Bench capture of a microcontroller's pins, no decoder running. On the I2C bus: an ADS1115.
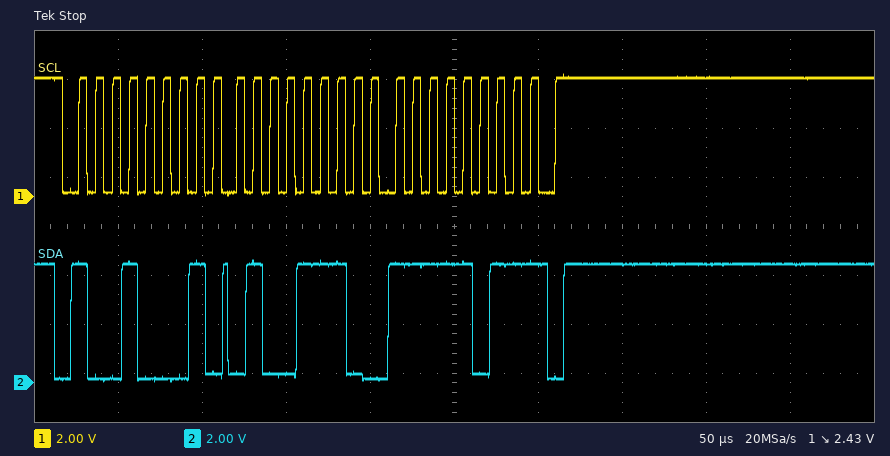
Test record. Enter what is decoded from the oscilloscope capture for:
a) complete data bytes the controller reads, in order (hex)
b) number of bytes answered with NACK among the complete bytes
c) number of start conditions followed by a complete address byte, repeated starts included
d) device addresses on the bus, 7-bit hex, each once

4E FB
1
1
0x48
